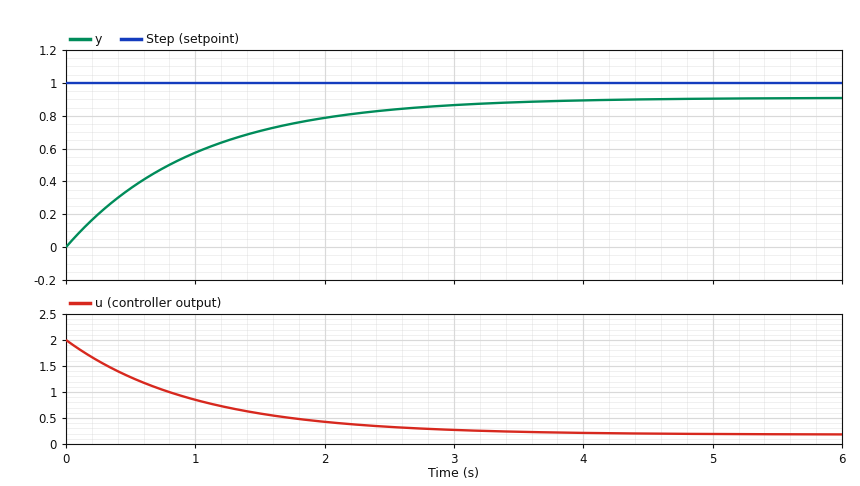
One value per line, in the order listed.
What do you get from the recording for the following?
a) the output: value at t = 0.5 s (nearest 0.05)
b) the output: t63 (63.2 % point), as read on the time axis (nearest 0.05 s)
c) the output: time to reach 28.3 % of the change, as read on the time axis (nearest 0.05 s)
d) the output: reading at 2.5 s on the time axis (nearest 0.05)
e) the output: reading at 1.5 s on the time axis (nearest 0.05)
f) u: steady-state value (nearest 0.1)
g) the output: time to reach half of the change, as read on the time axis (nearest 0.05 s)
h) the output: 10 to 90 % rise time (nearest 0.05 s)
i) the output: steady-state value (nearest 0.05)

0.35
1.00 s
0.35 s
0.85
0.70
0.2
0.70 s
2.20 s
0.90
